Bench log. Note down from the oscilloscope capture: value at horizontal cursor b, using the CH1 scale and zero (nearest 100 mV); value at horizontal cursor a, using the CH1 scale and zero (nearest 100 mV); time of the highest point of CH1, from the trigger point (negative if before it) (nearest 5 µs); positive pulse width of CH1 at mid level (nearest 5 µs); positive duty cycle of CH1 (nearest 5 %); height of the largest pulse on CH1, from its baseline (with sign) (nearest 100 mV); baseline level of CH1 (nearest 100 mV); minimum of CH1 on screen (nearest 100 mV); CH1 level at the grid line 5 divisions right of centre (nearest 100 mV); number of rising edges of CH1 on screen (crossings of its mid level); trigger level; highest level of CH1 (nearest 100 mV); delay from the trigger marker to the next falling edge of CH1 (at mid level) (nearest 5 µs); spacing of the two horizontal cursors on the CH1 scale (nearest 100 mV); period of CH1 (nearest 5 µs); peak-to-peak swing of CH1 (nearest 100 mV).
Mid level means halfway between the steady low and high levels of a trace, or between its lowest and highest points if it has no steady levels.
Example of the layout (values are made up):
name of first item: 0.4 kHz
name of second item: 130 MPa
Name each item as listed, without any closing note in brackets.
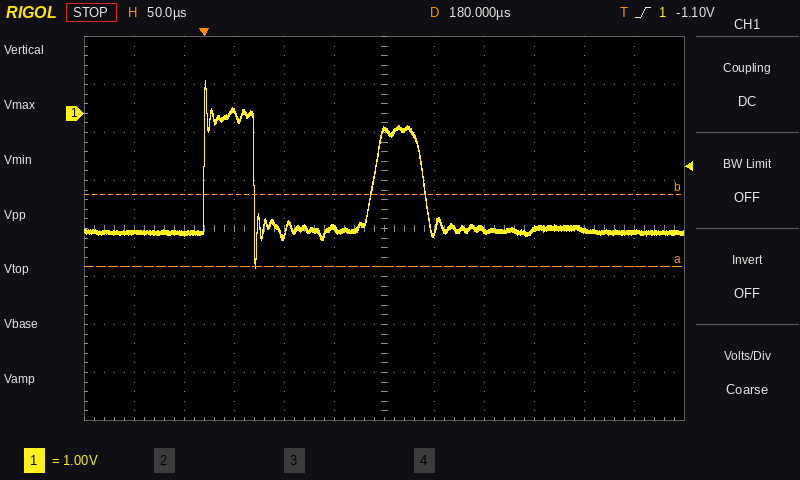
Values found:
value at horizontal cursor b, using the CH1 scale and zero: -1.7 V
value at horizontal cursor a, using the CH1 scale and zero: -3.2 V
time of the highest point of CH1, from the trigger point (negative if before it): 0 µs
positive pulse width of CH1 at mid level: 50 µs
positive duty cycle of CH1: 30 %
height of the largest pulse on CH1, from its baseline (with sign): +3.2 V
baseline level of CH1: -2.5 V
minimum of CH1 on screen: -3.2 V
CH1 level at the grid line 5 divisions right of centre: -2.5 V
number of rising edges of CH1 on screen: 2
trigger level: -1.10 V
highest level of CH1: 700 mV
delay from the trigger marker to the next falling edge of CH1 (at mid level): 50 µs
spacing of the two horizontal cursors on the CH1 scale: 1.5 V
period of CH1: 170 µs
peak-to-peak swing of CH1: 3.9 V
